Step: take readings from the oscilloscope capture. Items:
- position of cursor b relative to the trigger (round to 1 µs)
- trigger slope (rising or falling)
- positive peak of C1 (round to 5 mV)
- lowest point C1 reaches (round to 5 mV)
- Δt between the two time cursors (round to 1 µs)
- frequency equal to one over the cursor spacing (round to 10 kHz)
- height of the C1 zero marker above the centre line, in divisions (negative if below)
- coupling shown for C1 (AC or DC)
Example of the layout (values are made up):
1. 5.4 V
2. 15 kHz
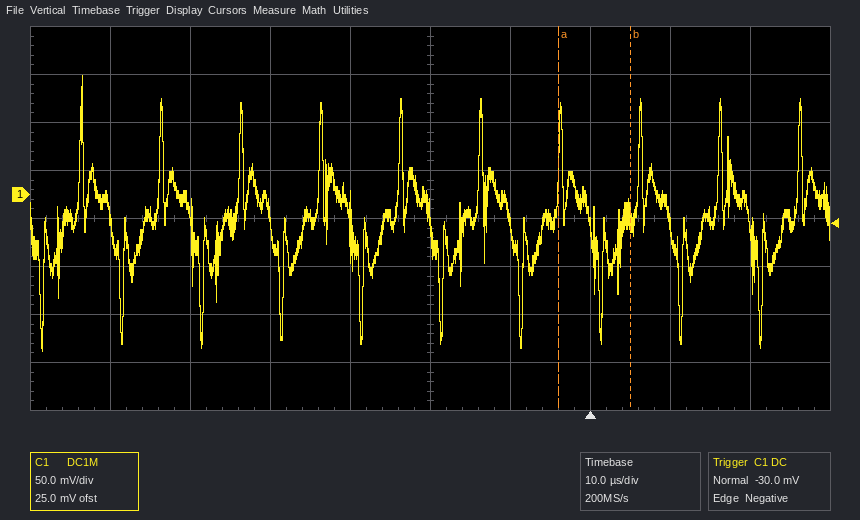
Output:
1. +5 µs
2. falling
3. 125 mV
4. -165 mV
5. 9 µs
6. 110 kHz
7. +0.5 div
8. DC
